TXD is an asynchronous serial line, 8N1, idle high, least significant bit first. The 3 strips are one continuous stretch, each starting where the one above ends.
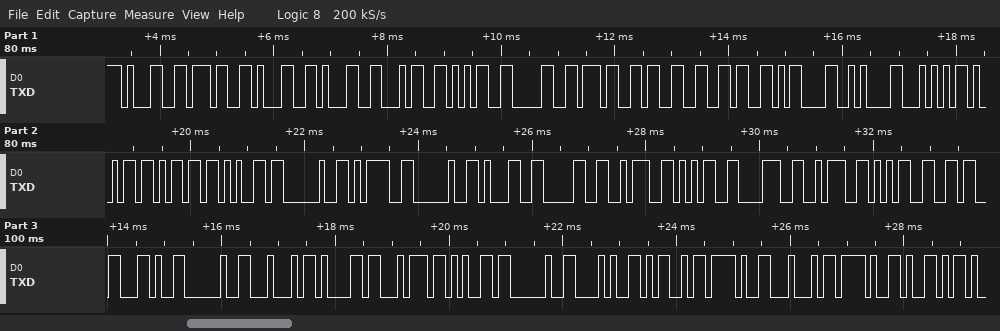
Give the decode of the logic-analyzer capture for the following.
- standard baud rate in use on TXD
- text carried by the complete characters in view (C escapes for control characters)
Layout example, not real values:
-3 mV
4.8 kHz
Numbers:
9600 baud
"1711450736\r\nTime = 10:58:56, Date (M/D/Y"
